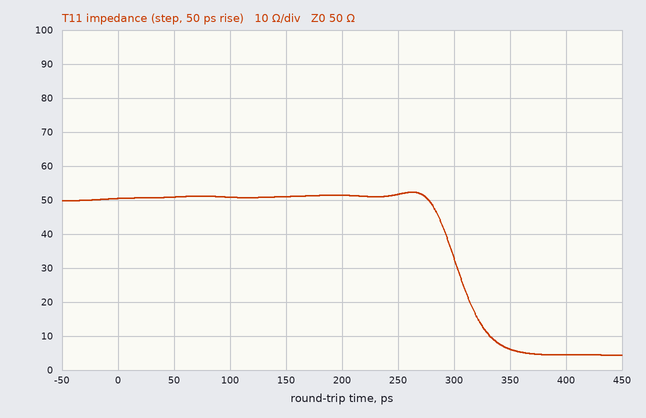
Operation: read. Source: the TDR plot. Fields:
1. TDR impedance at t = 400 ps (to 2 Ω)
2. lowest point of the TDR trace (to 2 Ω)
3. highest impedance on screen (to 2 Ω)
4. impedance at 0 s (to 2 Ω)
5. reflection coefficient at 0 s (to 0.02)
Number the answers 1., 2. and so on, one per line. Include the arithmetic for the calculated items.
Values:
1. 4 Ω
2. 4 Ω
3. 52 Ω
4. 50 Ω
5. (50 − 50)/(50 + 50) ≈ 0.00
